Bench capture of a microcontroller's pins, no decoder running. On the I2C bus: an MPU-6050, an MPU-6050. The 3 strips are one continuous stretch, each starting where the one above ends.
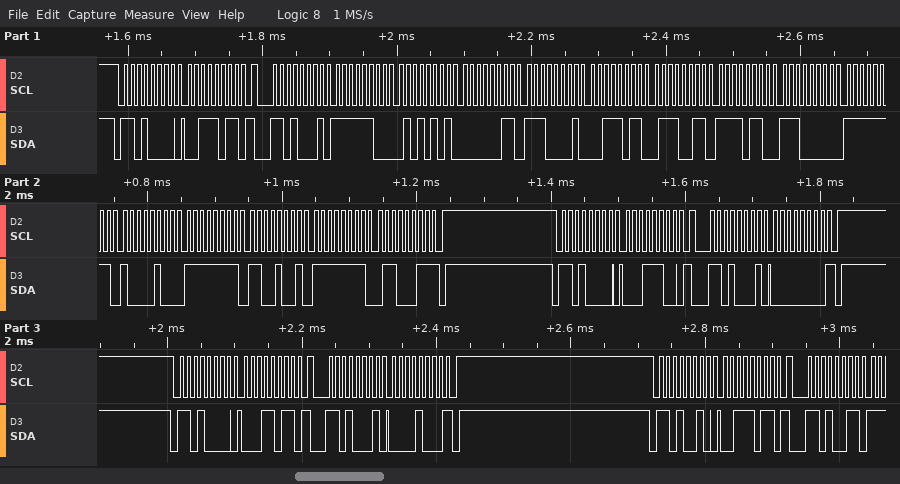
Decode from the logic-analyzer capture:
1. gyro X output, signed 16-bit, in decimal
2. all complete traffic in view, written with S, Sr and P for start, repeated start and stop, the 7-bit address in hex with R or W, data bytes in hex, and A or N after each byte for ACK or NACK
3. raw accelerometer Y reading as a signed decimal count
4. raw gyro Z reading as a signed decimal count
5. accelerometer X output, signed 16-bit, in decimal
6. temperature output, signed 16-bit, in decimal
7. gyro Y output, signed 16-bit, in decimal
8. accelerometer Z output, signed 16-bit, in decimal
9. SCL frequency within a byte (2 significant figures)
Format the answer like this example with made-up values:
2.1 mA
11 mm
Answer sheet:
-124
S 68W A 3B A Sr 68R A FC A 55 A 03 A E1 A 3B A 73 A F6 A E0 A FF A 84 A FF A C9 A FF A 63 N P S 68W A 1C A Sr 68R A 00 N P S 68W A 1B A Sr 68R A 08 N P S 69W A 3B A Sr 69R A
993
-157
-939
-2336
-55
15219
100 kHz
